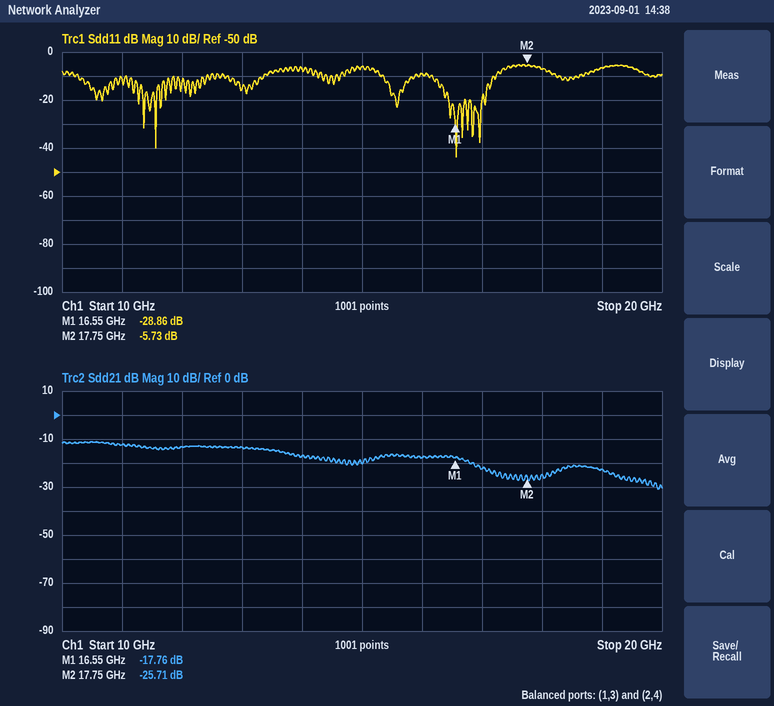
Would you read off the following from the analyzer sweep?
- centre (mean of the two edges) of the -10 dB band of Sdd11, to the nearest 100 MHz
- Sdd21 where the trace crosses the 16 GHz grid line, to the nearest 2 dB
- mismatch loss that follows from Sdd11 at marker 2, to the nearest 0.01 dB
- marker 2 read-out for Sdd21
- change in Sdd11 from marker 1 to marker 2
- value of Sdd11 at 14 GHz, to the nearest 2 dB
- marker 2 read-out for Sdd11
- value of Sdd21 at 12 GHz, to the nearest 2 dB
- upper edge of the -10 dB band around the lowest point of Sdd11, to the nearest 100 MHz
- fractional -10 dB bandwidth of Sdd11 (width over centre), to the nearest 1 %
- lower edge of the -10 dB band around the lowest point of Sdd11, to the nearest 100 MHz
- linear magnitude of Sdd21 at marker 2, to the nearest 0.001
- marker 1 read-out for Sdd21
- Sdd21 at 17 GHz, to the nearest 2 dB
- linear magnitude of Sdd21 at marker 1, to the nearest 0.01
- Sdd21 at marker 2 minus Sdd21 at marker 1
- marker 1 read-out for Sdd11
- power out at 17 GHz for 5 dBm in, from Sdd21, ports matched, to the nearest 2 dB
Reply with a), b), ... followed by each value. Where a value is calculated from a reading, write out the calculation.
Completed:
a) 16.7 GHz
b) -18 dB
c) −10 log10(1 − 10^(-5.73/10)) ≈ 1.35 dB
d) -25.71 dB
e) -5.73 − (-28.86) = 23.13 dB
f) -8 dB
g) -5.73 dB
h) -14 dB
i) 17.2 GHz
j) 1 GHz / 16.7 GHz ≈ 6 %
k) 16.2 GHz
l) 10^(-25.71/20) ≈ 0.052
m) -17.76 dB
n) -22 dB
o) 10^(-17.76/20) ≈ 0.13
p) -25.71 − (-17.76) = -7.95 dB
q) -28.86 dB
r) 5 dBm + (-22 dB) = -18 dBm
